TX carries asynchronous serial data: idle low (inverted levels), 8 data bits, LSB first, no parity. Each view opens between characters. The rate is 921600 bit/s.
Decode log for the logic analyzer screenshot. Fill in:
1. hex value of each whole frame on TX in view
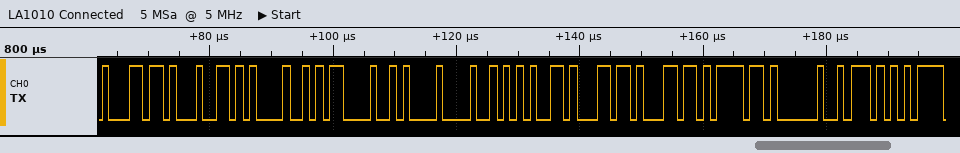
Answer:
27, 37, BD, E5, EB, 6F, 35, 27, 27, 21, BF, 51
